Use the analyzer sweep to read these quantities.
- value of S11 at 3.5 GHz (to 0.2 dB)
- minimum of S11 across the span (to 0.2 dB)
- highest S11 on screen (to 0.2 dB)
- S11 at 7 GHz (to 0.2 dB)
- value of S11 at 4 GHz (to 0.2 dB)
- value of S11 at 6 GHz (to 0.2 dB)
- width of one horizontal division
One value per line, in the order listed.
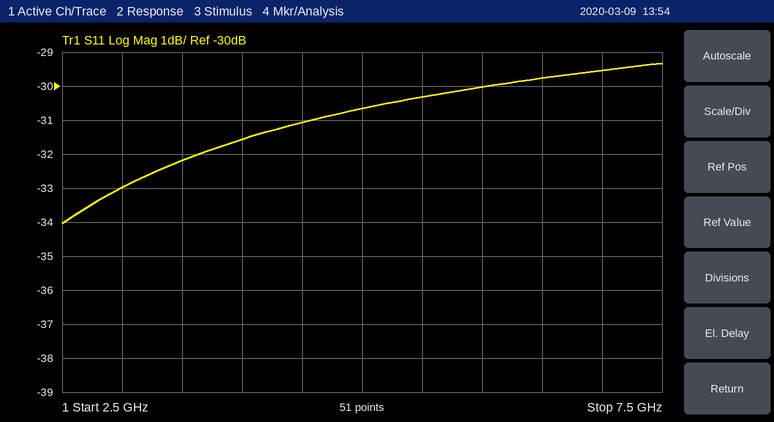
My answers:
-32.2 dB
-34.0 dB
-29.4 dB
-29.6 dB
-31.6 dB
-30.0 dB
500 MHz
